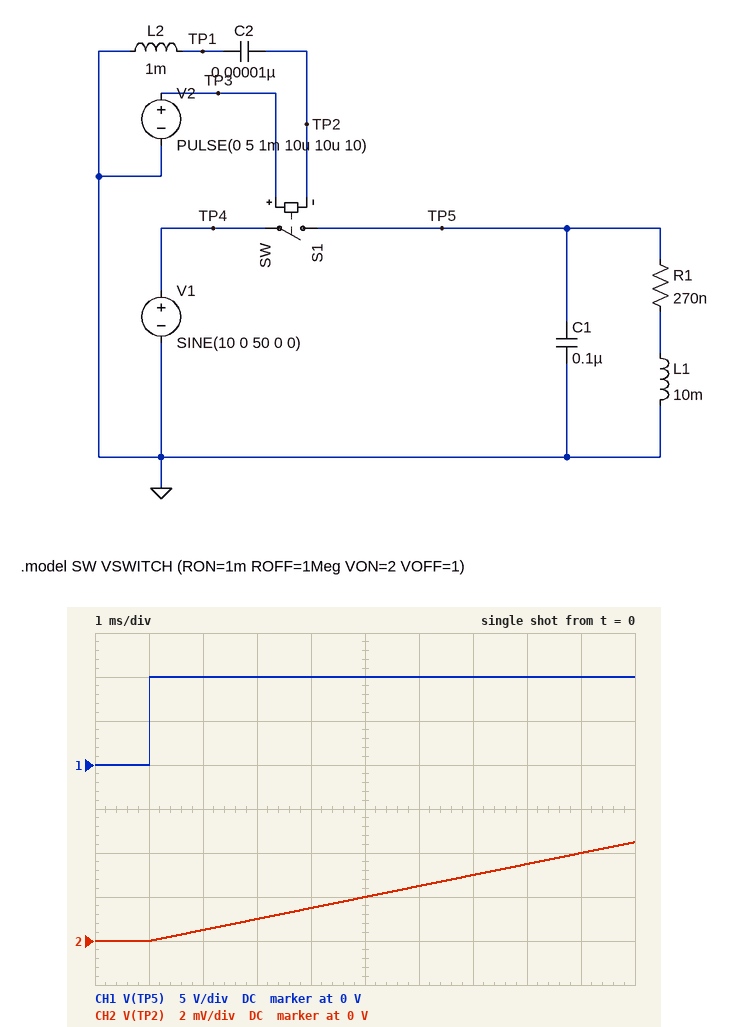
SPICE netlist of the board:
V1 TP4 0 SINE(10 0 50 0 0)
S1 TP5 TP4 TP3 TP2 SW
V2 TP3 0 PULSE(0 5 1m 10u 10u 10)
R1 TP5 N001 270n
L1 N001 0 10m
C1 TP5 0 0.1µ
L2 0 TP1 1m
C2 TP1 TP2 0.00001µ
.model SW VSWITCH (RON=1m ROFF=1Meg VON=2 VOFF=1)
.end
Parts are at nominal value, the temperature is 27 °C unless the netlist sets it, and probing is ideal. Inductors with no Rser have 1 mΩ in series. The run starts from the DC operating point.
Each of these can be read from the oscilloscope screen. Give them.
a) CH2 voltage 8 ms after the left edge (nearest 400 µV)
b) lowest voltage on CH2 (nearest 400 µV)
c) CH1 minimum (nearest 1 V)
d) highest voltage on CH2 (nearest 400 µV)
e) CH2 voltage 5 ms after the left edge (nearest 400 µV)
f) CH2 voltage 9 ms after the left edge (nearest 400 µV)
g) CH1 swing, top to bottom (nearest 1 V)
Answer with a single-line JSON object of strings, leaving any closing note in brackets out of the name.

{"CH2 voltage 8 ms after the left edge": "3.6 mV", "lowest voltage on CH2": "0 V", "CH1 minimum": "0 V", "highest voltage on CH2": "4.4 mV", "CH2 voltage 5 ms after the left edge": "2.0 mV", "CH2 voltage 9 ms after the left edge": "4.0 mV", "CH1 swing, top to bottom": "10 V"}
